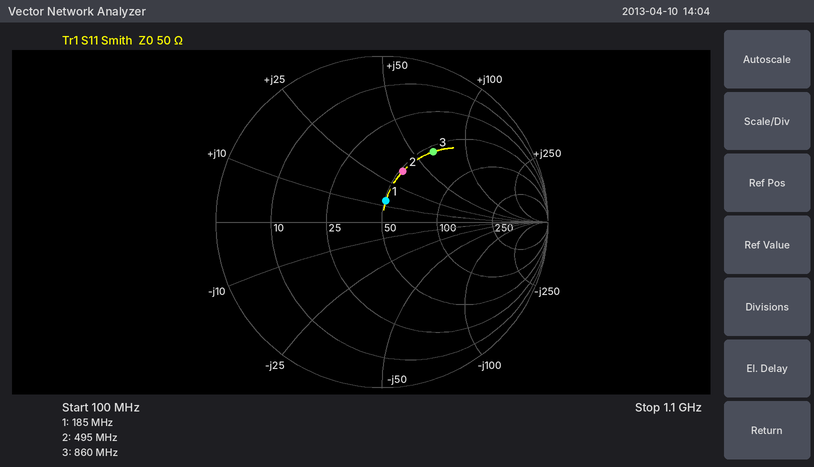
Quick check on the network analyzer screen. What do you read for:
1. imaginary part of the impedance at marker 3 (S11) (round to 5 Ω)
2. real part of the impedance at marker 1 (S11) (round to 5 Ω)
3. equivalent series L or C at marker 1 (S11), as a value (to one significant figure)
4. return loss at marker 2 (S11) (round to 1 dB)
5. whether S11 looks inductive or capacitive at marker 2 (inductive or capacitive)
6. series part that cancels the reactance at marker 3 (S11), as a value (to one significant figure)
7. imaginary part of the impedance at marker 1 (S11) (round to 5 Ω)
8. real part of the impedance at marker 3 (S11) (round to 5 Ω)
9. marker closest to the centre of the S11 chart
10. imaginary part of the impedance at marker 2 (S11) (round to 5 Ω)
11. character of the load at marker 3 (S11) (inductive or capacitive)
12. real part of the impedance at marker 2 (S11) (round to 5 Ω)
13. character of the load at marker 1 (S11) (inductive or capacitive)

+65 Ω
50 Ω
10 nH
10 dB
inductive
3 pF
+15 Ω
55 Ω
marker 1
+35 Ω
inductive
50 Ω
inductive
